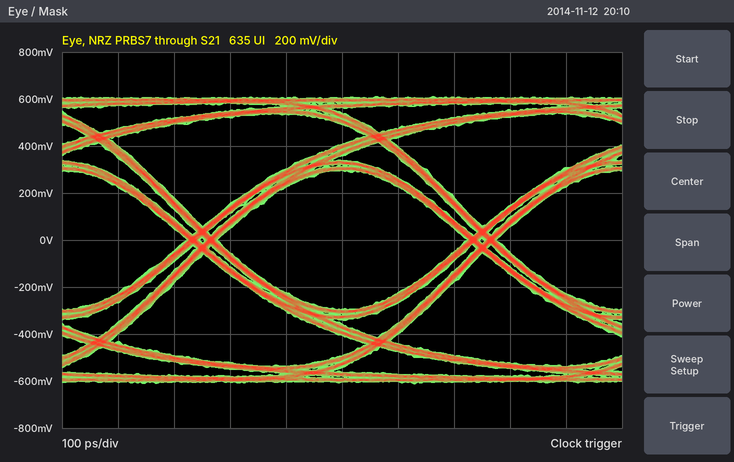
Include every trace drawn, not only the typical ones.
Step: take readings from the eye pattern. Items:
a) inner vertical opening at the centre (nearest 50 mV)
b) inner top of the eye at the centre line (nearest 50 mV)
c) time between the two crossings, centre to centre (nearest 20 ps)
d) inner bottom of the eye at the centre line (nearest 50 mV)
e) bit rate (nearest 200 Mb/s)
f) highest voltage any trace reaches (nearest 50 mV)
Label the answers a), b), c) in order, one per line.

a) 600 mV
b) 300 mV
c) 500 ps
d) -300 mV
e) 2.0 Gb/s
f) 600 mV
